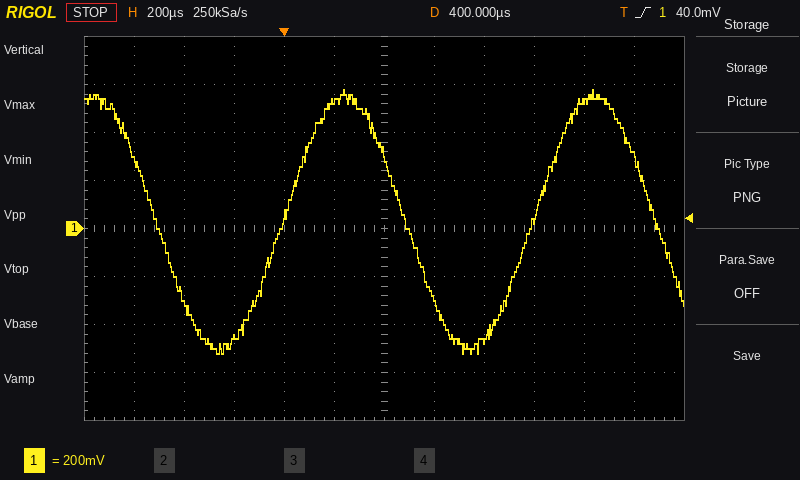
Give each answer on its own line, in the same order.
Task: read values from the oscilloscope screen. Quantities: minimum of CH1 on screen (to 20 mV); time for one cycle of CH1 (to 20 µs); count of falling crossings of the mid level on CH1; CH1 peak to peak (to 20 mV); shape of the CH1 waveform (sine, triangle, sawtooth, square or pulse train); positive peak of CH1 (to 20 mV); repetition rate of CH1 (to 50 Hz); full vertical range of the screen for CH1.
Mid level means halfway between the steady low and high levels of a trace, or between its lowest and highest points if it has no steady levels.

-520 mV
1.00 ms
3
1.10 V
sine
580 mV
1.00 kHz
1.6 V
